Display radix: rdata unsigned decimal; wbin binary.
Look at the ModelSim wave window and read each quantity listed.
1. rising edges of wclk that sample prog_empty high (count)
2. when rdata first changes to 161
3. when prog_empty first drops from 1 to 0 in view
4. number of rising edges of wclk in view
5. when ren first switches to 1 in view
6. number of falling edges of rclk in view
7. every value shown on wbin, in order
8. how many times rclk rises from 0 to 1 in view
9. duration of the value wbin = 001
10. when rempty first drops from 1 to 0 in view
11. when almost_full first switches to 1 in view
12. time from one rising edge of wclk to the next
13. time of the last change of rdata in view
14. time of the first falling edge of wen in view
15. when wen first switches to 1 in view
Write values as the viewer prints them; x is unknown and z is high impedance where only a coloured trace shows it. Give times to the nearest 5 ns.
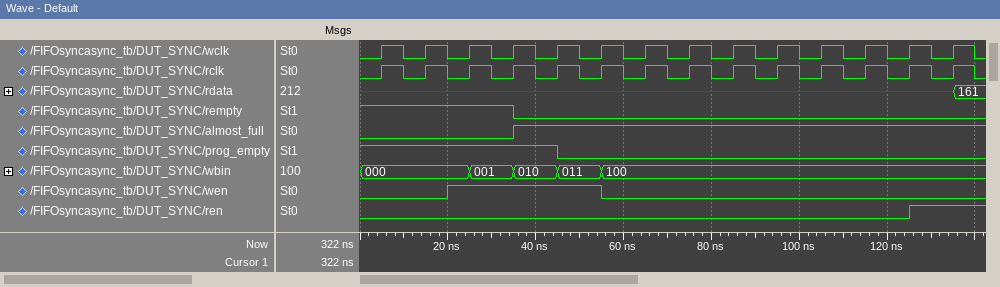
5
135 ns
45 ns
14
125 ns
14
000, 001, 010, 011, 100
14
10 ns
35 ns
35 ns
10 ns
135 ns
55 ns
20 ns
